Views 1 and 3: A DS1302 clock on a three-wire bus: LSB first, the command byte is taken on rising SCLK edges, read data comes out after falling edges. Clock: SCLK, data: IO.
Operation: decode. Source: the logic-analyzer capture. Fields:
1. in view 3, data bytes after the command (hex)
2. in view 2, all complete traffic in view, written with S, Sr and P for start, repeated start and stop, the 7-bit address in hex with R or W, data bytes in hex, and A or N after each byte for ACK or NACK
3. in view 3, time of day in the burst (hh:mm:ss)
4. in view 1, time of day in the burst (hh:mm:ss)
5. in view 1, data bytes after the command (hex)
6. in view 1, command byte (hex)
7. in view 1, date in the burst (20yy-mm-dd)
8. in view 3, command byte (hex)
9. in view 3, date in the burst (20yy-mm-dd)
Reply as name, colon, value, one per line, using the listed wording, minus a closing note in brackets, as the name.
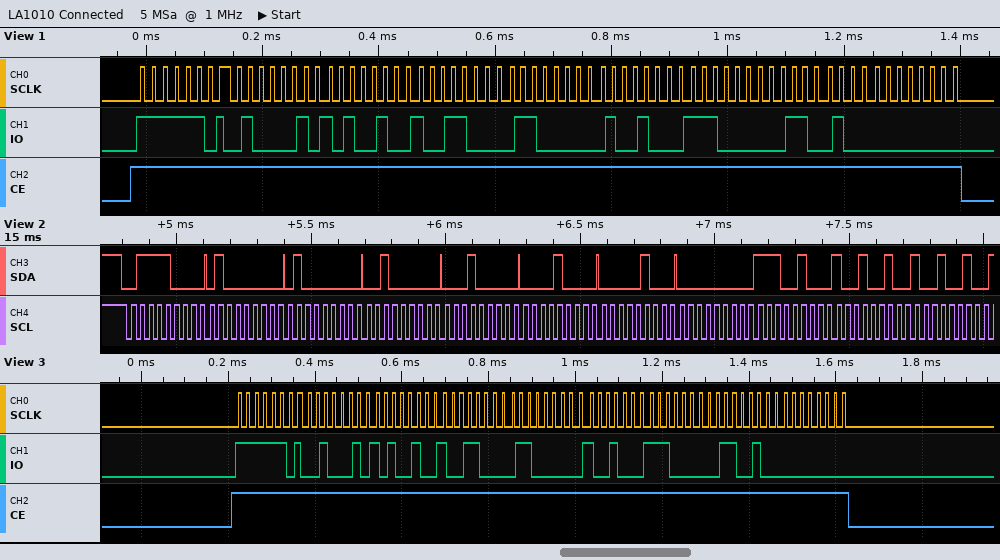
in view 3, data bytes after the command: 44 25 19 06 12 07 26 00
in view 2, all complete traffic in view, written with S, Sr and P for start, repeated start and stop, the 7-bit address in hex with R or W, data bytes in hex, and A or N after each byte for ACK or NACK: S 3CW A 40 A 40 A 20 A 10 A 08 A 04 A 00 A E4 A 92 A 92 A
in view 3, time of day in the burst: 19:25:44
in view 1, time of day in the burst: 19:25:42
in view 1, data bytes after the command: 42 25 19 06 12 07 26 00
in view 1, command byte: 0xBF
in view 1, date in the burst: 2026-12-06
in view 3, command byte: 0xBF
in view 3, date in the burst: 2026-12-06
